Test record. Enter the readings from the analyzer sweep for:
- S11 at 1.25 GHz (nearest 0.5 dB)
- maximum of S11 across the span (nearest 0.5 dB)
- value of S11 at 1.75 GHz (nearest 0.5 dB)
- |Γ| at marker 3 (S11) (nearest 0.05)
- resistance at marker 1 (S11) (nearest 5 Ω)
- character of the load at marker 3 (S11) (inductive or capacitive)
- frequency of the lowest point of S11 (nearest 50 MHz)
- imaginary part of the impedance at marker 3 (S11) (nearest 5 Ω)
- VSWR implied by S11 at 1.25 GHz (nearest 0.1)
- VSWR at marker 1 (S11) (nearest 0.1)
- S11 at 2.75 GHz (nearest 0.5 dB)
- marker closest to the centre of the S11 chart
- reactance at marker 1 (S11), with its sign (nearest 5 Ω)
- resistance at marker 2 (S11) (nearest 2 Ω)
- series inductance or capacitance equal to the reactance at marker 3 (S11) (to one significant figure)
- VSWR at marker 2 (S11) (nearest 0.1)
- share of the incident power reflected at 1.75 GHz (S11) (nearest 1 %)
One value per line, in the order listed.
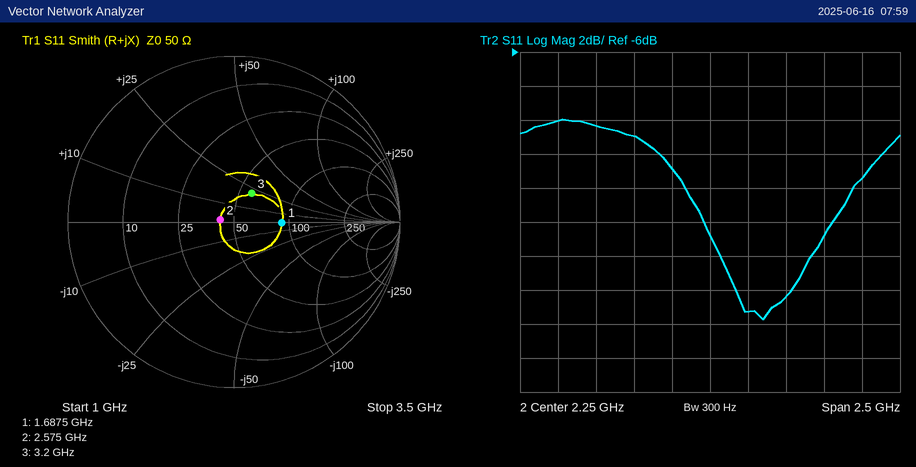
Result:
-10.0 dB
-10.0 dB
-11.0 dB
0.20
90 Ω
inductive
2.60 GHz
+20 Ω
1.9
1.8
-20.5 dB
marker 2
0 Ω
42 Ω
1 nH
1.2
8 %
